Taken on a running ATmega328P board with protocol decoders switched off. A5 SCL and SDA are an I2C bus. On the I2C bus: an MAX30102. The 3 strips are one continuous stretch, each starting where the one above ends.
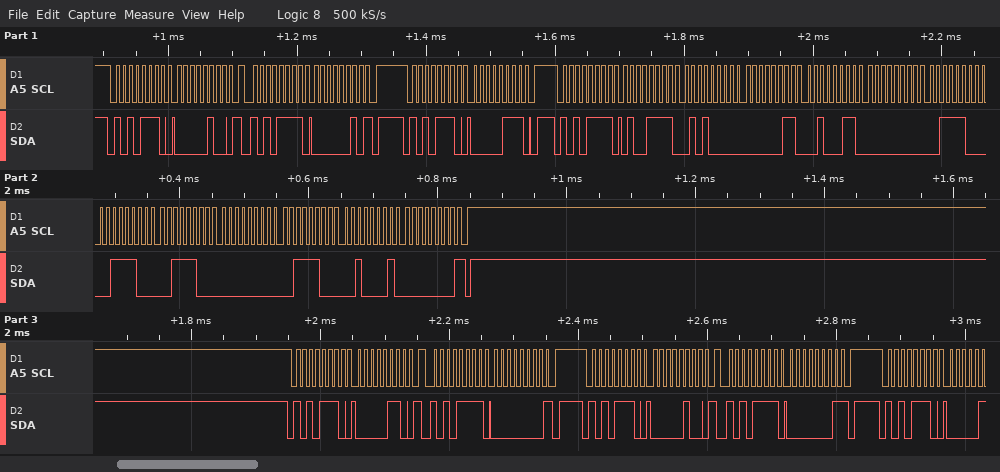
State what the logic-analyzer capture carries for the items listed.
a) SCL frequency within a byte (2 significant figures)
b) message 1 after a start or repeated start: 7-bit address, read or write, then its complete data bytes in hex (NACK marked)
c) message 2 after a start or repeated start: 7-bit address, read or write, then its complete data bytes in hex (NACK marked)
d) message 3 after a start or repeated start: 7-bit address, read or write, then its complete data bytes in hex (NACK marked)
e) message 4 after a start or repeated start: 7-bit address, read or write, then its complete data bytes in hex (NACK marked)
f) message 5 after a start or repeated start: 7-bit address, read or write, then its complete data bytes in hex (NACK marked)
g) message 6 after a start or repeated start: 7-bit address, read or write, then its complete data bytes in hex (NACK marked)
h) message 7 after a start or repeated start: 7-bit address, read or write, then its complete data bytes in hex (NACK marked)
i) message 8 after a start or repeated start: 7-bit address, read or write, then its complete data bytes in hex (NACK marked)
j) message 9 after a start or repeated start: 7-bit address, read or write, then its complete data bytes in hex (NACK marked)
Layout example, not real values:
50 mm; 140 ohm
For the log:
100 kHz; 0x57 write: 04; 0x57 read: 02 NACK; 0x57 write: 07; 0x57 read: 4F 50 03 23 00 3C 3C 3C 00 3C 21 00 NACK; 0x57 write: 06; 0x57 read: 00 NACK; 0x57 write: 04; 0x57 read: 01 NACK; 0x57 write
